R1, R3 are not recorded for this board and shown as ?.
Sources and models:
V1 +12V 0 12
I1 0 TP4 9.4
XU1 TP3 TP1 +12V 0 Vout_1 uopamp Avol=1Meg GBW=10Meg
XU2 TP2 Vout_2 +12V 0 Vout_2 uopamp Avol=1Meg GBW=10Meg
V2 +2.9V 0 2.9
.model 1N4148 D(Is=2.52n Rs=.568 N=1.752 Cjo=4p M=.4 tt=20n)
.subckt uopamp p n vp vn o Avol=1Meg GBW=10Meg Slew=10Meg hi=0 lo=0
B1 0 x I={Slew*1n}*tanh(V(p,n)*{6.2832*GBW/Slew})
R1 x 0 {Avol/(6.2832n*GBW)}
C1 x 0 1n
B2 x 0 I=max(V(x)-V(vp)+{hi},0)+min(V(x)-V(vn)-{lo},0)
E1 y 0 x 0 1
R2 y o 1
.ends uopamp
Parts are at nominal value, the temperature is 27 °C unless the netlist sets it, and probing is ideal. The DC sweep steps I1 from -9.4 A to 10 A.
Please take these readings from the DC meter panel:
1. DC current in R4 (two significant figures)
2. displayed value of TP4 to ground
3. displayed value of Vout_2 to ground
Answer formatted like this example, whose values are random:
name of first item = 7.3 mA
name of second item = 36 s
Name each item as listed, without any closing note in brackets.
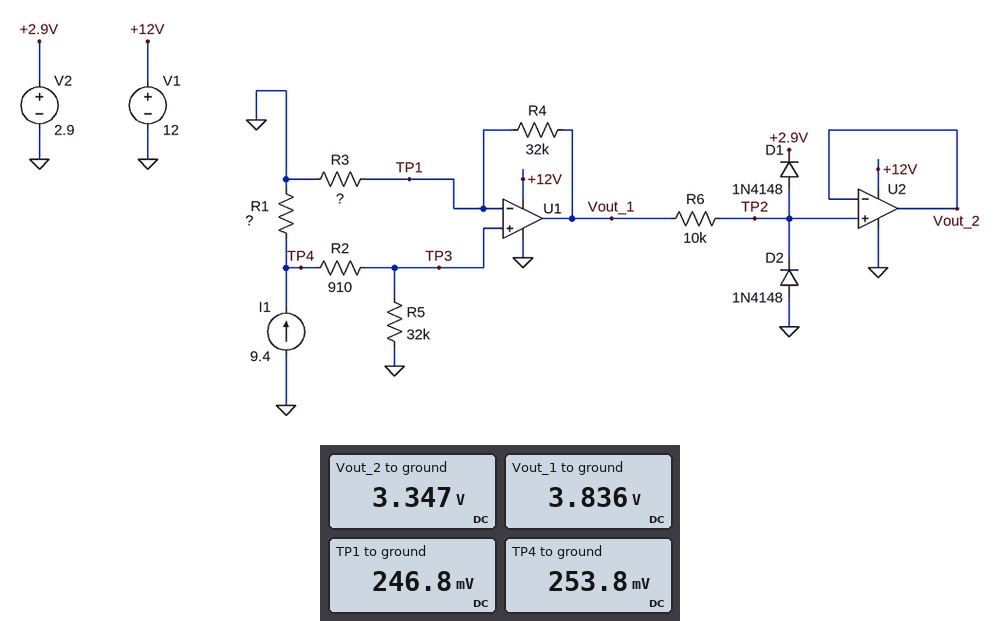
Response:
DC current in R4 = 110 µA
displayed value of TP4 to ground = 253.8 mV
displayed value of Vout_2 to ground = 3.347 V
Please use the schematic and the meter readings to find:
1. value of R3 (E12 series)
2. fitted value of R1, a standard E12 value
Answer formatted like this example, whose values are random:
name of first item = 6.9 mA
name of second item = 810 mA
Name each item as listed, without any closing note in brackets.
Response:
value of R3 = 2.2 kΩ
fitted value of R1, a standard E12 value = 0.027 Ω
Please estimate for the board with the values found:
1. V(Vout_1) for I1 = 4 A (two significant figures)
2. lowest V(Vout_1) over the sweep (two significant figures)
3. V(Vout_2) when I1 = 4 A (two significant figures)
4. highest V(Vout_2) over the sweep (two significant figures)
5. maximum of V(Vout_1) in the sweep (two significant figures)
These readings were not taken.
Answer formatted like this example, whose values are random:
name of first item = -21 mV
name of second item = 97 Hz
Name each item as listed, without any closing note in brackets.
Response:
V(Vout_1) for I1 = 4 A = 1.6 V
lowest V(Vout_1) over the sweep = -9.1 mV
V(Vout_2) when I1 = 4 A = 1.6 V
highest V(Vout_2) over the sweep = 3.4 V
maximum of V(Vout_1) in the sweep = 4.1 V
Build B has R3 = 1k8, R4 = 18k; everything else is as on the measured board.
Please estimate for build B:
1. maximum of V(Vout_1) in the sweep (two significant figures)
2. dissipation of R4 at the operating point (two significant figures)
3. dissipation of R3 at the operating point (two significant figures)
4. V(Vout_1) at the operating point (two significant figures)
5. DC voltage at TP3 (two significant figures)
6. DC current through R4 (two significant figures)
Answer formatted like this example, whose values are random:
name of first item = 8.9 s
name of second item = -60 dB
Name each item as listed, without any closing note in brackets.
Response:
maximum of V(Vout_1) in the sweep = 2.9 V
dissipation of R4 at the operating point = 340 µW
dissipation of R3 at the operating point = 34 µW
V(Vout_1) at the operating point = 2.7 V
DC voltage at TP3 = 250 mV
DC current through R4 = 140 µA
